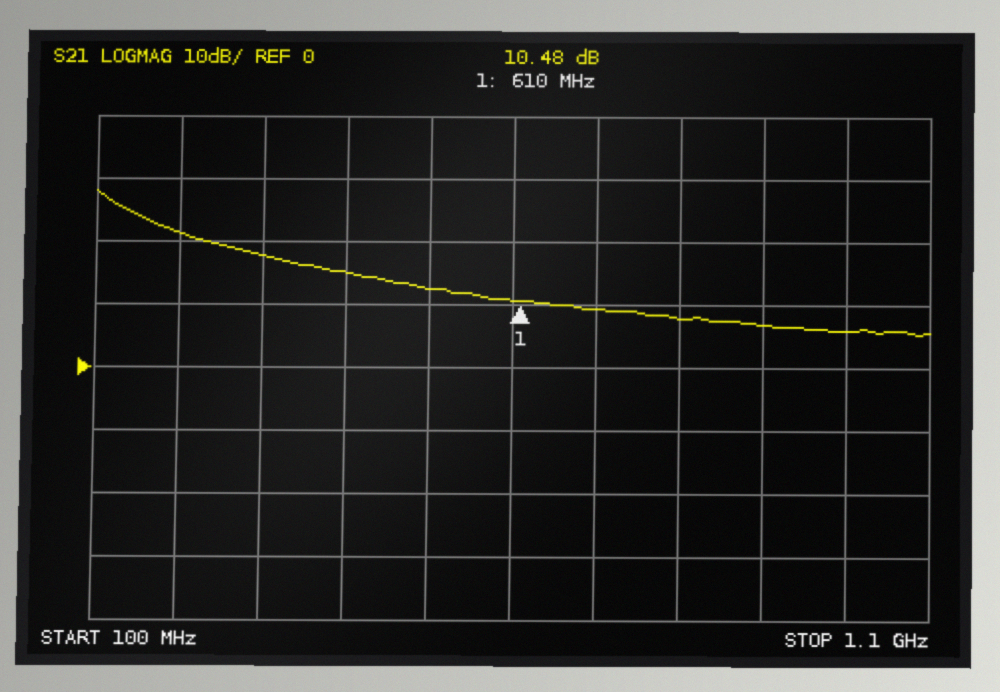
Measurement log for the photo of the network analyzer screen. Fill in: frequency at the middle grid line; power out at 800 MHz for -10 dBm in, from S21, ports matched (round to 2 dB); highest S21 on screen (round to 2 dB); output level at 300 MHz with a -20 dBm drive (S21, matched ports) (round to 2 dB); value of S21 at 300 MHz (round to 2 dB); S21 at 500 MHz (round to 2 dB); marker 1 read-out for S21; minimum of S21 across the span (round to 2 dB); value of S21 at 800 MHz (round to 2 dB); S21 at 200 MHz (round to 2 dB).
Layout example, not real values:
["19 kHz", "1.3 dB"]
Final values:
["600 MHz", "-2 dBm", "28 dB", "-2 dBm", "18 dB", "12 dB", "10.48 dB", "6 dB", "8 dB", "22 dB"]
